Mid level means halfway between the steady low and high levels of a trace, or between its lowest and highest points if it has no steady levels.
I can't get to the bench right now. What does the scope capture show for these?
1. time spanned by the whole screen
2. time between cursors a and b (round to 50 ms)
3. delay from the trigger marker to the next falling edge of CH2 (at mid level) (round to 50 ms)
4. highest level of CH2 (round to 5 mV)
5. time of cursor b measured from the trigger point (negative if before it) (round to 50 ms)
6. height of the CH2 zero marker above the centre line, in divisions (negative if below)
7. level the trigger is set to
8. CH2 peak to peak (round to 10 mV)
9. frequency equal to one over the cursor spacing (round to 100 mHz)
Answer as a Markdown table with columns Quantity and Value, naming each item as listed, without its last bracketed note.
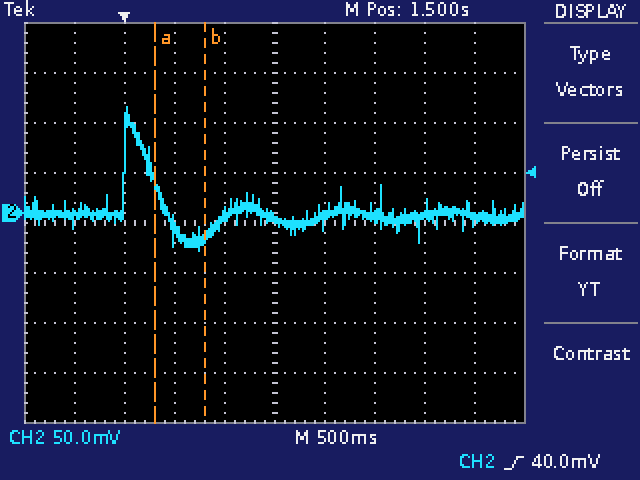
| Quantity | Value |
|---|---|
| time spanned by the whole screen | 5 s |
| time between cursors a and b | 500 ms |
| delay from the trigger marker to the next falling edge of CH2 (at mid level) | 300 ms |
| highest level of CH2 | 105 mV |
| time of cursor b measured from the trigger point (negative if before it) | +800 ms |
| height of the CH2 zero marker above the centre line, in divisions | +0.2 div |
| level the trigger is set to | 40.0 mV |
| CH2 peak to peak | 140 mV |
| frequency equal to one over the cursor spacing | 2.0 Hz |
